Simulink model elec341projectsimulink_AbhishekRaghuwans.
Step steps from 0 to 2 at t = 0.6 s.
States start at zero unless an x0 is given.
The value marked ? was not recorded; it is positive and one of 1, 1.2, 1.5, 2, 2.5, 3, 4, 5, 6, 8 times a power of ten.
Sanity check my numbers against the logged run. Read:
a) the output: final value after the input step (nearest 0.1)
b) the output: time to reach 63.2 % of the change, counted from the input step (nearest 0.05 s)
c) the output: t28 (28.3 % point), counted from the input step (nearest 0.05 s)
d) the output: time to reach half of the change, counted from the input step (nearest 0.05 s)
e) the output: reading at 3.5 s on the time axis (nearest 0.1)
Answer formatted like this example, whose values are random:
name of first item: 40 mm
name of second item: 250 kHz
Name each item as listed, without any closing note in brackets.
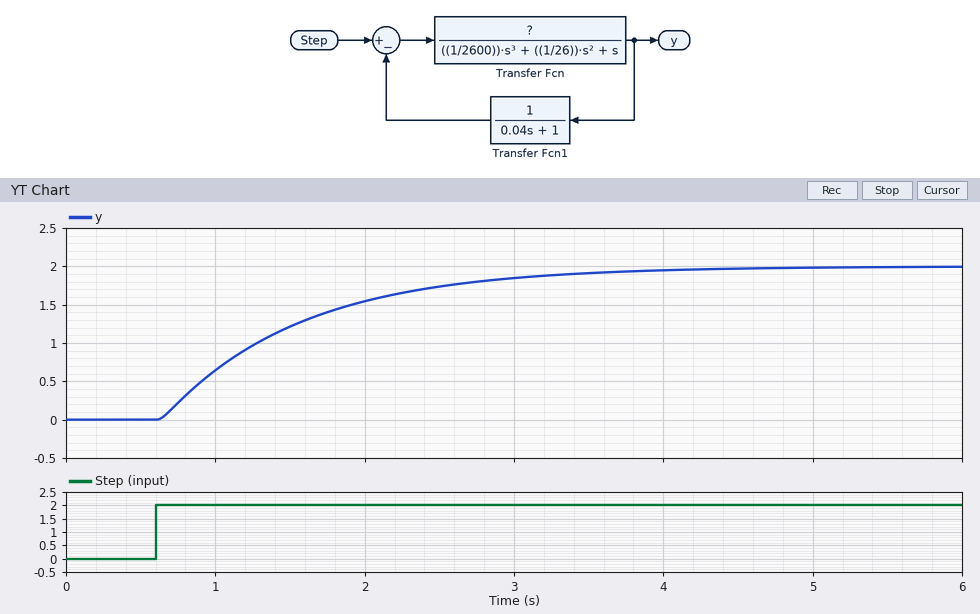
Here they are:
the output: final value after the input step: 2.0
the output: time to reach 63.2 % of the change, counted from the input step: 0.95 s
the output: t28 (28.3 % point), counted from the input step: 0.35 s
the output: time to reach half of the change, counted from the input step: 0.70 s
the output: reading at 3.5 s on the time axis: 1.9
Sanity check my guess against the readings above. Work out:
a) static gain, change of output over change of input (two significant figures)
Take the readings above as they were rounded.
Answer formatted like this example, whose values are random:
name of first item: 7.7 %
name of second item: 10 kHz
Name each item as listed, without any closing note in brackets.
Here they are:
static gain, change of output over change of input: 1.0
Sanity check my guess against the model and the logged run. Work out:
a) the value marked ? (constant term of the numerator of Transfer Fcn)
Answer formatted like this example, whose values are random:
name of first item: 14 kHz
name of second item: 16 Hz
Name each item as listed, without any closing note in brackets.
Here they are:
the value marked ?: 1
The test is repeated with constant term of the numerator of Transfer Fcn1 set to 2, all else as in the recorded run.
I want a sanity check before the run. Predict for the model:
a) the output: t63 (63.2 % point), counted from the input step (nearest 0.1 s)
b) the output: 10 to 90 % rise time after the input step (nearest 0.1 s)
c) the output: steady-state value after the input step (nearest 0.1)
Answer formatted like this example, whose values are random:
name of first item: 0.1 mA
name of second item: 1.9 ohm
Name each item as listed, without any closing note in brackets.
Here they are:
the output: t63 (63.2 % point), counted from the input step: 0.5 s
the output: 10 to 90 % rise time after the input step: 0.9 s
the output: steady-state value after the input step: 1.0
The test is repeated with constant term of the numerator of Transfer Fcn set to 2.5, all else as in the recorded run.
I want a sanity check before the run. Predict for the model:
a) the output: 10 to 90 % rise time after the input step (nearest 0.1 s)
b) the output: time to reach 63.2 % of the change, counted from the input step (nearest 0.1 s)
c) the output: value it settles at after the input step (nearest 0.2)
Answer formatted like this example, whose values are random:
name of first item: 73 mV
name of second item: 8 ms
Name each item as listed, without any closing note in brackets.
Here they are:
the output: 10 to 90 % rise time after the input step: 0.7 s
the output: time to reach 63.2 % of the change, counted from the input step: 0.4 s
the output: value it settles at after the input step: 2.0
